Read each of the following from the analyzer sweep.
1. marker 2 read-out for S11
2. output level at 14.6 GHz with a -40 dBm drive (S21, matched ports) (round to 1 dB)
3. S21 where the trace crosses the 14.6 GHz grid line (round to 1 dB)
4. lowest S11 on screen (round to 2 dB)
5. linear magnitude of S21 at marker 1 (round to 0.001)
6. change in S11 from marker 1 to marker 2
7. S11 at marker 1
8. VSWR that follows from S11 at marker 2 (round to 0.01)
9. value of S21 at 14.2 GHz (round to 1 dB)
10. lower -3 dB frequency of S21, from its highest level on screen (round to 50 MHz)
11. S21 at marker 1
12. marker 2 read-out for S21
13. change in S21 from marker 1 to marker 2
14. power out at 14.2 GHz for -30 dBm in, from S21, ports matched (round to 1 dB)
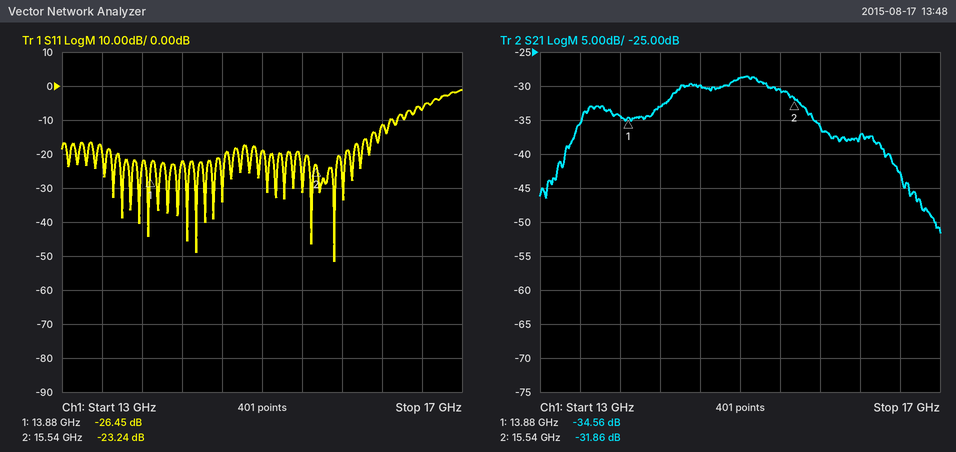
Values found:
-23.24 dB
-70 dBm
-30 dB
-52 dB
0.019
3.21 dB
-26.45 dB
1.15
-33 dB
14.30 GHz
-34.56 dB
-31.86 dB
2.70 dB
-63 dBm
